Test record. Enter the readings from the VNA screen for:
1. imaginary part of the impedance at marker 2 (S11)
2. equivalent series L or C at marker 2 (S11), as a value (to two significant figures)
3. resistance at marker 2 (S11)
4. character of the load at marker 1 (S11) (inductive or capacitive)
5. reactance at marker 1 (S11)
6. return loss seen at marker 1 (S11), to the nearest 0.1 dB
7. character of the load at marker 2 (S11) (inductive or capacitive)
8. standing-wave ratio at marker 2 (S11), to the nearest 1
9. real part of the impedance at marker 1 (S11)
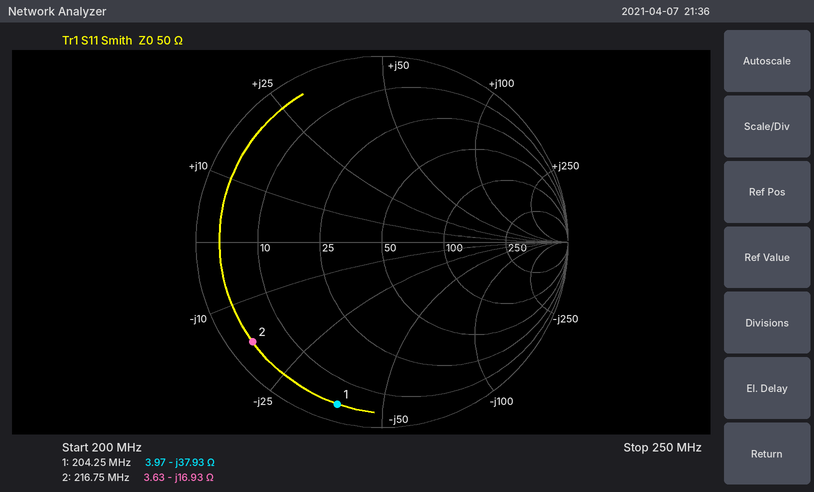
-16.93 Ω
43 pF
3.63 Ω
capacitive
-37.93 Ω
0.9 dB
capacitive
15
3.97 Ω
